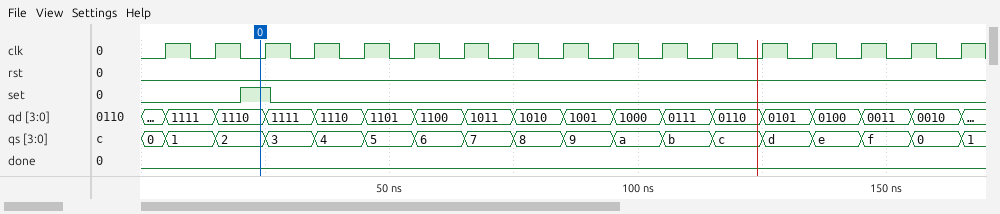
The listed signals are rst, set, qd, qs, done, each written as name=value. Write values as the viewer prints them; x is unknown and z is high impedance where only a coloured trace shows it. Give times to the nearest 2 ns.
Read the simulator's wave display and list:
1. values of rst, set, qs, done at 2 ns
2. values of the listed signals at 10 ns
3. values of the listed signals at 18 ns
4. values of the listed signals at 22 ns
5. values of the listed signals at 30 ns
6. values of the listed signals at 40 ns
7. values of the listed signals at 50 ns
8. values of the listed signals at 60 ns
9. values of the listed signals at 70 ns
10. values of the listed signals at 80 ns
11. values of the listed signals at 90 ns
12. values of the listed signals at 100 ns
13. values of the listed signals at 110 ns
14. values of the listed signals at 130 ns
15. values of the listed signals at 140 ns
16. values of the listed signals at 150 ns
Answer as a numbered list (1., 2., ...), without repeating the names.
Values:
1. rst=0, set=0, qs=0, done=0
2. rst=0, set=0, qd=1111, qs=1, done=0
3. rst=0, set=0, qd=1110, qs=2, done=0
4. rst=0, set=1, qd=1110, qs=2, done=0
5. rst=0, set=0, qd=1111, qs=3, done=0
6. rst=0, set=0, qd=1110, qs=4, done=0
7. rst=0, set=0, qd=1101, qs=5, done=0
8. rst=0, set=0, qd=1100, qs=6, done=0
9. rst=0, set=0, qd=1011, qs=7, done=0
10. rst=0, set=0, qd=1010, qs=8, done=0
11. rst=0, set=0, qd=1001, qs=9, done=0
12. rst=0, set=0, qd=1000, qs=a, done=0
13. rst=0, set=0, qd=0111, qs=b, done=0
14. rst=0, set=0, qd=0101, qs=d, done=0
15. rst=0, set=0, qd=0100, qs=e, done=0
16. rst=0, set=0, qd=0011, qs=f, done=0
